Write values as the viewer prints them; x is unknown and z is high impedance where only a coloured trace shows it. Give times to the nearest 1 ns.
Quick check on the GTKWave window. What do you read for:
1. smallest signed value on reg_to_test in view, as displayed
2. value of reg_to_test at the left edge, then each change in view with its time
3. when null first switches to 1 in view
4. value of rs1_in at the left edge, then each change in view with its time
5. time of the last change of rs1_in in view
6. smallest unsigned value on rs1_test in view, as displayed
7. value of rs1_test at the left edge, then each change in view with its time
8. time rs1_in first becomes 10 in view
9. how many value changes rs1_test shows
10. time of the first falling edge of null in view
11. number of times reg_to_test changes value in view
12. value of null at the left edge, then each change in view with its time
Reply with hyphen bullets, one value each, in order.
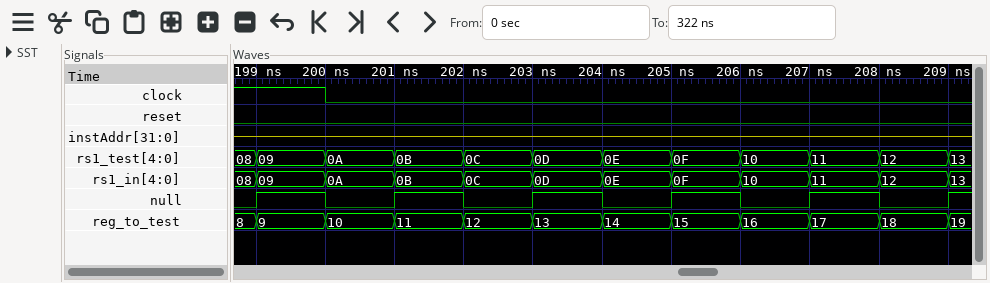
- 8
- 8, 9 at 199 ns, 10 at 200 ns, 11 at 201 ns, 12 at 202 ns, 13 at 203 ns, 14 at 204 ns, 15 at 205 ns, 16 at 206 ns, 17 at 207 ns, 18 at 208 ns, 19 at 209 ns
- 199 ns
- 08, 09 at 199 ns, 0A at 200 ns, 0B at 201 ns, 0C at 202 ns, 0D at 203 ns, 0E at 204 ns, 0F at 205 ns, 10 at 206 ns, 11 at 207 ns, 12 at 208 ns, 13 at 209 ns
- 209 ns
- 08
- 08, 09 at 199 ns, 0A at 200 ns, 0B at 201 ns, 0C at 202 ns, 0D at 203 ns, 0E at 204 ns, 0F at 205 ns, 10 at 206 ns, 11 at 207 ns, 12 at 208 ns, 13 at 209 ns
- 206 ns
- 11
- 200 ns
- 11
- 0, 1 at 199 ns, 0 at 200 ns, 1 at 201 ns, 0 at 202 ns, 1 at 203 ns, 0 at 204 ns, 1 at 205 ns, 0 at 206 ns, 1 at 207 ns, 0 at 208 ns, 1 at 209 ns
